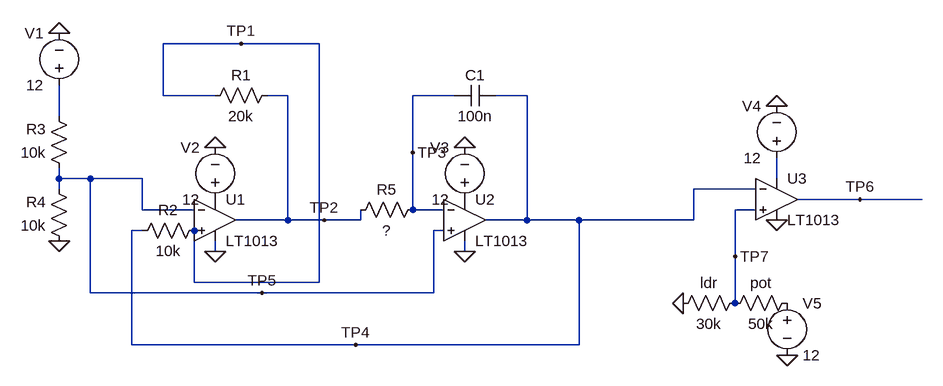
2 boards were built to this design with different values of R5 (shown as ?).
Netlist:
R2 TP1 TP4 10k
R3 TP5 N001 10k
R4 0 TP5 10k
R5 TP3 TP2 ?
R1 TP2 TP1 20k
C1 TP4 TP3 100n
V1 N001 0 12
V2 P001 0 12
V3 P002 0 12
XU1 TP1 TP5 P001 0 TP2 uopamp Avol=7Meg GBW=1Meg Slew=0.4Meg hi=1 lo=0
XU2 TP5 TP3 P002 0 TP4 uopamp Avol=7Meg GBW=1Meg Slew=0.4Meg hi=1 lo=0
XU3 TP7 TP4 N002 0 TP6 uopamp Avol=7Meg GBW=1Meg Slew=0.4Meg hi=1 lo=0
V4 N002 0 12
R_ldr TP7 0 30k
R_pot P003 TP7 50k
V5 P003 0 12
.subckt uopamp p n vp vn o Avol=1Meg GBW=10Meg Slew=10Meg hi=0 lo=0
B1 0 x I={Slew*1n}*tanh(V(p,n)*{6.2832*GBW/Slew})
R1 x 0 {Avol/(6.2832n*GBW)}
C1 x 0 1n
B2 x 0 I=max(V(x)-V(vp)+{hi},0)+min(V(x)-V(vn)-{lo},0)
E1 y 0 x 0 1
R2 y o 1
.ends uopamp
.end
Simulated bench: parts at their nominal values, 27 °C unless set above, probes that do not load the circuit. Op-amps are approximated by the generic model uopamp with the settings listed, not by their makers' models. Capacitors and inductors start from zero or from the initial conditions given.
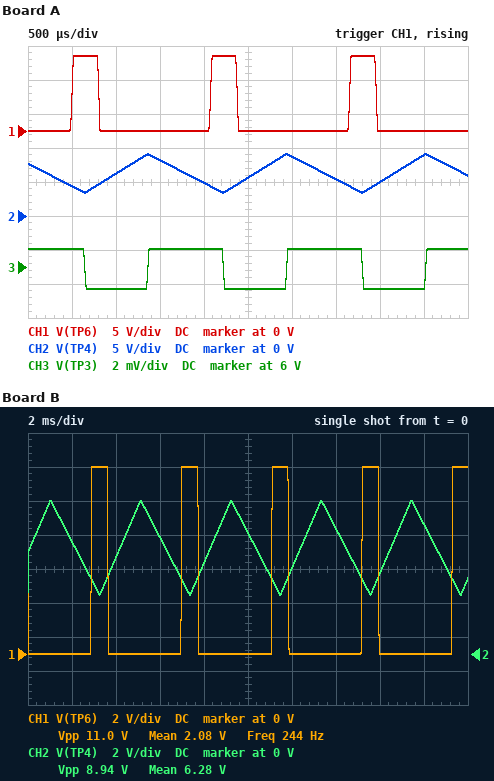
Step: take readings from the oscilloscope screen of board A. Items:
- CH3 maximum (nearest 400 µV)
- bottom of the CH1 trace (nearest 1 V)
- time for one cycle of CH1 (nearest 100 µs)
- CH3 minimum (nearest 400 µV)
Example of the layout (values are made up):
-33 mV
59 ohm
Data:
6.0012 V
0 V
1.6 ms
5.9988 V
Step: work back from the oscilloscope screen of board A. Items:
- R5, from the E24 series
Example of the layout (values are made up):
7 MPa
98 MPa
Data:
7.5 kΩ
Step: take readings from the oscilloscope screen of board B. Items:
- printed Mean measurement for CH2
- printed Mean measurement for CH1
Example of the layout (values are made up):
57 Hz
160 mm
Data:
6.28 V
2.08 V
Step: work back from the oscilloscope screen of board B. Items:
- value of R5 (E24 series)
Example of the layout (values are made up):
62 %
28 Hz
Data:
20 kΩ
